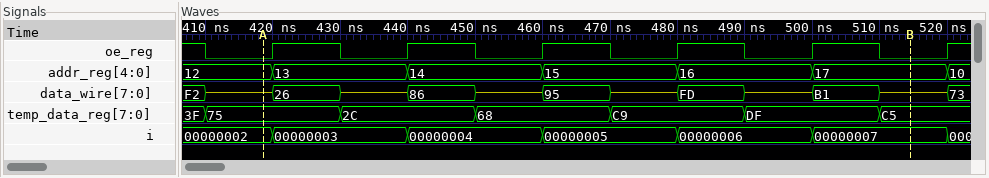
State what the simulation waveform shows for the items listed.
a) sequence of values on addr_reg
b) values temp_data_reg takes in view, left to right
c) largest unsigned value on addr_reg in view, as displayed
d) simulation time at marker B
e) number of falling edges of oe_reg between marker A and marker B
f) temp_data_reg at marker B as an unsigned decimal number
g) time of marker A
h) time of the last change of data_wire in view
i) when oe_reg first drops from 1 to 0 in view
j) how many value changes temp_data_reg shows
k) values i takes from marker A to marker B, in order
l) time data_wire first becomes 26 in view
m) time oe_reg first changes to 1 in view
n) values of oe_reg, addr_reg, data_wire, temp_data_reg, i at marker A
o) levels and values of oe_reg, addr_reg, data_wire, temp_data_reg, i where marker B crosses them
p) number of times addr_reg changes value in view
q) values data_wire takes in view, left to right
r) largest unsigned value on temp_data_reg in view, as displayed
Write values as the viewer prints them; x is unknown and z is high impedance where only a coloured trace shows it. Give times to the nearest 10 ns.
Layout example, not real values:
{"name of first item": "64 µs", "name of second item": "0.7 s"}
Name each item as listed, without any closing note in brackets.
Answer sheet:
{"sequence of values on addr_reg": "12, 13, 14, 15, 16, 17, 10", "values temp_data_reg takes in view, left to right": "3F, 75, 2C, 68, C9, DF, C5", "largest unsigned value on addr_reg in view, as displayed": "17", "simulation time at marker B": "510 ns", "number of falling edges of oe_reg between marker A and marker B": "5", "temp_data_reg at marker B as an unsigned decimal number": "197", "time of marker A": "420 ns", "time of the last change of data_wire in view": "520 ns", "when oe_reg first drops from 1 to 0 in view": "410 ns", "how many value changes temp_data_reg shows": "6", "values i takes from marker A to marker B, in order": "00000002, 00000003, 00000004, 00000005, 00000006, 00000007", "time data_wire first becomes 26 in view": "420 ns", "time oe_reg first changes to 1 in view": "420 ns", "values of oe_reg, addr_reg, data_wire, temp_data_reg, i at marker A": "oe_reg=0, addr_reg=12, data_wire=z, temp_data_reg=75, i=00000002", "levels and values of oe_reg, addr_reg, data_wire, temp_data_reg, i where marker B crosses them": "oe_reg=0, addr_reg=17, data_wire=z, temp_data_reg=C5, i=00000007", "number of times addr_reg changes value in view": "6", "values data_wire takes in view, left to right": "F2, z, 26, z, 86, z, 95, z, FD, z, B1, z, 73", "largest unsigned value on temp_data_reg in view, as displayed": "DF"}
